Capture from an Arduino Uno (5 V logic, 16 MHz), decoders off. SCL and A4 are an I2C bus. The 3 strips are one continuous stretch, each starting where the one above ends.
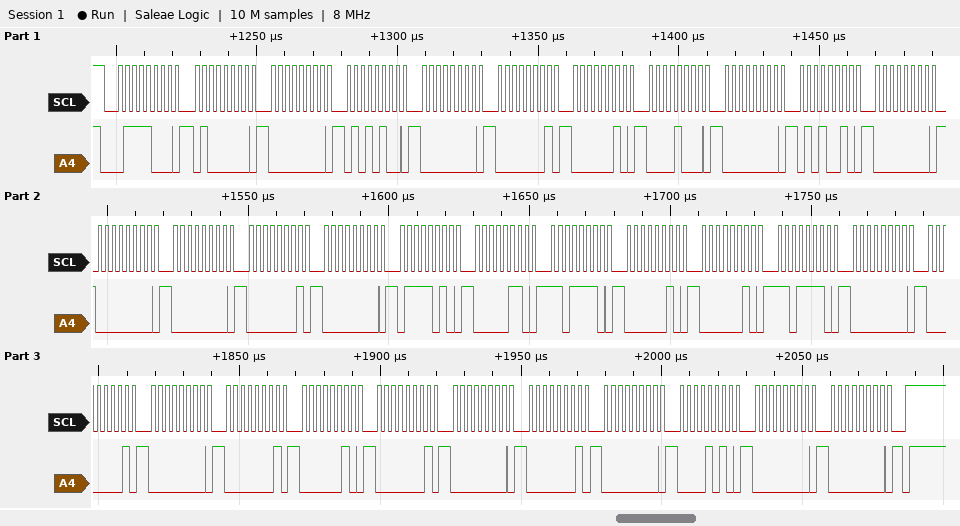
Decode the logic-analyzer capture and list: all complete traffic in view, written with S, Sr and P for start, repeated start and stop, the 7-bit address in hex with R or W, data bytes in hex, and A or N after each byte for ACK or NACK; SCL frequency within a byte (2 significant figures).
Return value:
S 3CW A 40 A 00 A 54 A 00 A 01 A 02 A 08 A 00 A 52 A 00 A 00 A 00 A 01 A 00 A 7A A 06 A DE A 02 A 02 A DE A 00 A 01 A 00 A 01 A 02 A 01 A 00 A 01 A 00 A 0A A 00 A 00 A P
400 kHz
